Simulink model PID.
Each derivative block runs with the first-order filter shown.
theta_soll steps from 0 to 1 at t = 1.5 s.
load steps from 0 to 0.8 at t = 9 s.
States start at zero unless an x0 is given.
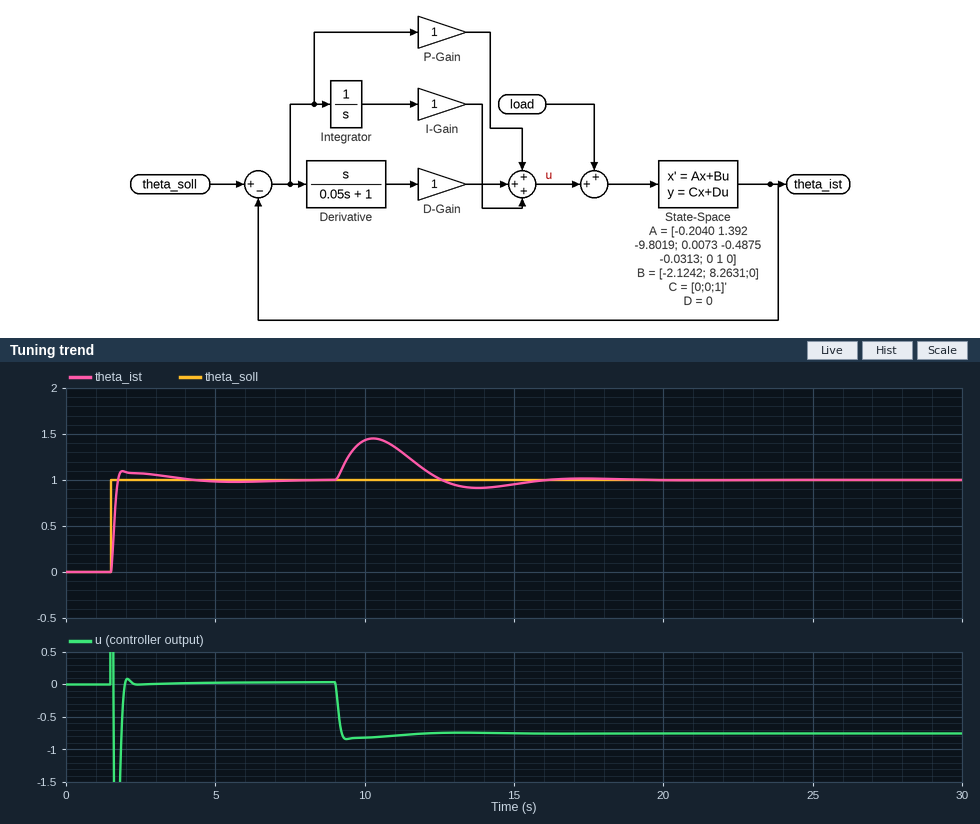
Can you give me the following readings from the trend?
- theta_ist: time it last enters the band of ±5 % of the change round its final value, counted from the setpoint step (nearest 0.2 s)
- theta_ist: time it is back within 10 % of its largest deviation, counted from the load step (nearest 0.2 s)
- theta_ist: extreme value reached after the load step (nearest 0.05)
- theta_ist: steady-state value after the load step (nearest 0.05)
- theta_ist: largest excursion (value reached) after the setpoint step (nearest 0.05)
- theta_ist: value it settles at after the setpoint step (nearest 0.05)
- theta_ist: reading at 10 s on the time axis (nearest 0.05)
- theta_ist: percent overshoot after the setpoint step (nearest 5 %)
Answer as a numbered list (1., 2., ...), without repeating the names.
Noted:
1. 1.6 s
2. 6.0 s
3. 1.45
4. 1.00
5. 1.10
6. 1.00
7. 1.45
8. 10 %
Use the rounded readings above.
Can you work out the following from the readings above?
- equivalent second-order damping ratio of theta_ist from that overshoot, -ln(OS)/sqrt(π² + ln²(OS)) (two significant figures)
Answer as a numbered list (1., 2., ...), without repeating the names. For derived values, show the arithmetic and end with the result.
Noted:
1. ln(0.1) = -2.303; 2.303 / sqrt(9.870 + 5.302) = 0.59
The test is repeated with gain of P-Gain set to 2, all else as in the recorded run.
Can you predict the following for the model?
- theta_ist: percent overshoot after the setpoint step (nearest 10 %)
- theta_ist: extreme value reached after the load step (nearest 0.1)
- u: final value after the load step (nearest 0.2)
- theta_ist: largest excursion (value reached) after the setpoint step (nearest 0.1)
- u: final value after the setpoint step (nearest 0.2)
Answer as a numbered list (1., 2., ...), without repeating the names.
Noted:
1. 20 %
2. 1.3
3. -0.8
4. 1.2
5. 0.0
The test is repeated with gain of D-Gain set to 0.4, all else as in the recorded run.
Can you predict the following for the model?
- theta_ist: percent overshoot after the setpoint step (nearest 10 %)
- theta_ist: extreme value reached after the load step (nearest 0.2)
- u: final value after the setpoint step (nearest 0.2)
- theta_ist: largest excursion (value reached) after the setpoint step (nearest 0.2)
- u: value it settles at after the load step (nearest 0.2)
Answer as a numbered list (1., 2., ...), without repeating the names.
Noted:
1. 30 %
2. 1.6
3. 0.0
4. 1.4
5. -0.8
